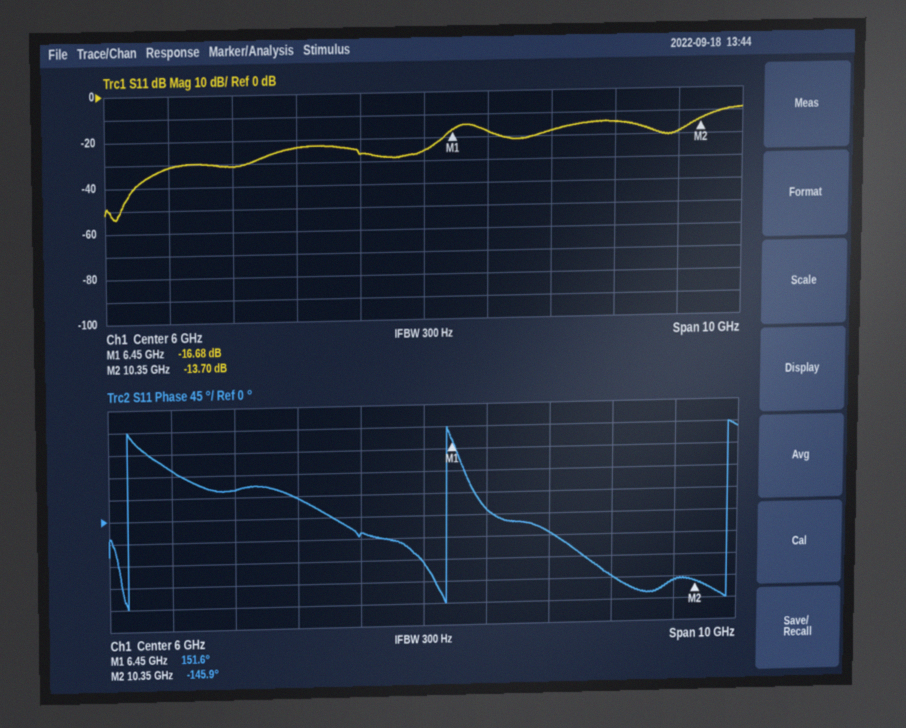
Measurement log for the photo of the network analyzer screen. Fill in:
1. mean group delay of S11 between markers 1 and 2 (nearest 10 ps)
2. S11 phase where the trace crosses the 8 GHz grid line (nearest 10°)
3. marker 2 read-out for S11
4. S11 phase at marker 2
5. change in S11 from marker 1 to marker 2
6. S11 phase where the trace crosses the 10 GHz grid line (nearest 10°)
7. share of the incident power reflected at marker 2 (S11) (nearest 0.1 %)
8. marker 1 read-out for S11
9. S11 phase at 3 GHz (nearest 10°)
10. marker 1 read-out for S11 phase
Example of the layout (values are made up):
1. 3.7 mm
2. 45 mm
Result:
1. 210 ps
2. -40°
3. -13.70 dB
4. -145.9°
5. 2.98 dB
6. -140°
7. 4.3 %
8. -16.68 dB
9. 60°
10. 151.6°
